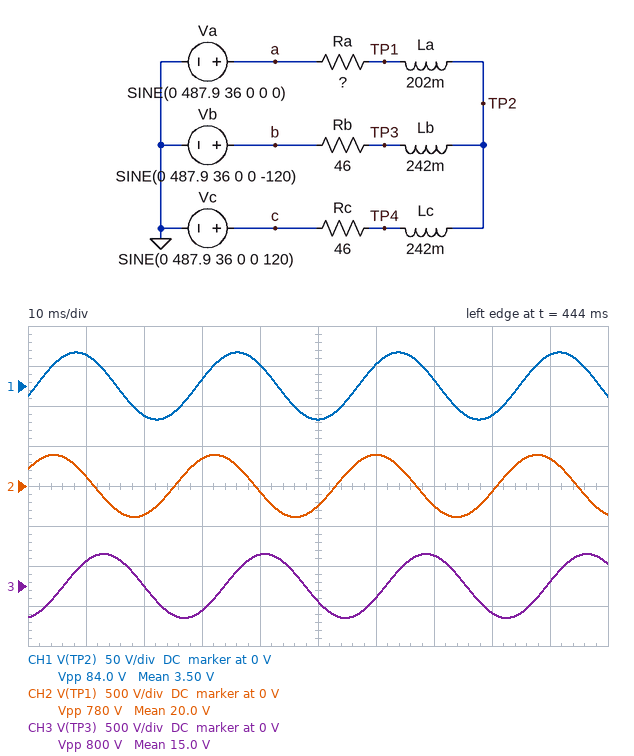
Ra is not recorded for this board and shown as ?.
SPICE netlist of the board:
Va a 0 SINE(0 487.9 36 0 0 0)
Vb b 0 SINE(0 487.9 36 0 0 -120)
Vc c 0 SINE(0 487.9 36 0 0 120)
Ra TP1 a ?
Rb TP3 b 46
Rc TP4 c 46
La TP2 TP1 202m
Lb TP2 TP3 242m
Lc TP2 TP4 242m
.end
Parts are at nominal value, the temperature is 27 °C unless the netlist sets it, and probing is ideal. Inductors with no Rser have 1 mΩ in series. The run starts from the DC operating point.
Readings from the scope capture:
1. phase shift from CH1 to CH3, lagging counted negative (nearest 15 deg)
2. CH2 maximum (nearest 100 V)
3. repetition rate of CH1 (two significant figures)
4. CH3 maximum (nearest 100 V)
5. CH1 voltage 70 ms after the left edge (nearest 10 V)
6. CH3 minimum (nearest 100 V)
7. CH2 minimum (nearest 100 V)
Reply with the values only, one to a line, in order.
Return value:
-60 deg
400 V
36 Hz
400 V
10 V
-400 V
-400 V
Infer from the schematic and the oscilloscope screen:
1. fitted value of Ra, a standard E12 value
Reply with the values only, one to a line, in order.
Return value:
33 Ω
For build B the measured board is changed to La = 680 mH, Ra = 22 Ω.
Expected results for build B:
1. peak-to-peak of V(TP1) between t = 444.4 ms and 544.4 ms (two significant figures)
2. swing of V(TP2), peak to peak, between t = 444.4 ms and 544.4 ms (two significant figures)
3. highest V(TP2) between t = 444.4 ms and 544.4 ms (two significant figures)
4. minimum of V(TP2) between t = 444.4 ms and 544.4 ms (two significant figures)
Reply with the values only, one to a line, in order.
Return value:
950 V
270 V
130 V
-130 V
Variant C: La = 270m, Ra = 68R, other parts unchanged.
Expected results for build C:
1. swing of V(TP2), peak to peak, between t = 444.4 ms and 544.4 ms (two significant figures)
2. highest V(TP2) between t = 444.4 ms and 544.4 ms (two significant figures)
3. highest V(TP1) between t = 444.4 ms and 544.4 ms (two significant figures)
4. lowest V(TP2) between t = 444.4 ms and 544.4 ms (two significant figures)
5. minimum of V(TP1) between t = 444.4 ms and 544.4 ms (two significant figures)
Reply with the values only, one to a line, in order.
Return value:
88 V
44 V
340 V
-44 V
-340 V
